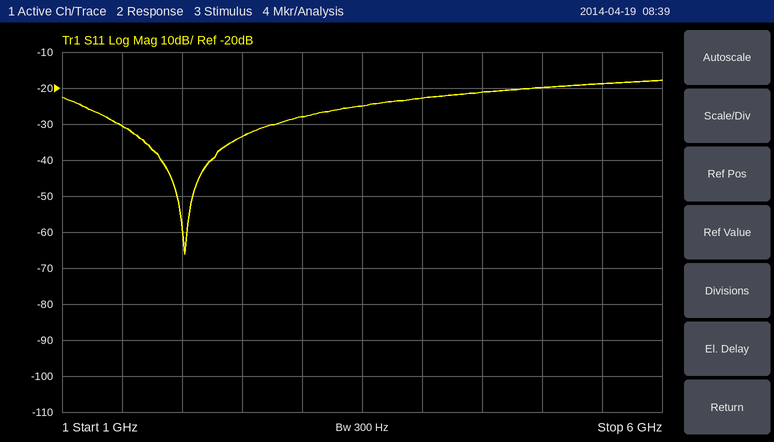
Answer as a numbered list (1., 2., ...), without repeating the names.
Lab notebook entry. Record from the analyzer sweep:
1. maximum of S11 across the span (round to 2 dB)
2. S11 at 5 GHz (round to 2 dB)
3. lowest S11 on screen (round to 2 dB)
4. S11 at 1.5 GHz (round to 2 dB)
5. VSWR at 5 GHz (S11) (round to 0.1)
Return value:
1. -18 dB
2. -20 dB
3. -66 dB
4. -30 dB
5. 1.2
